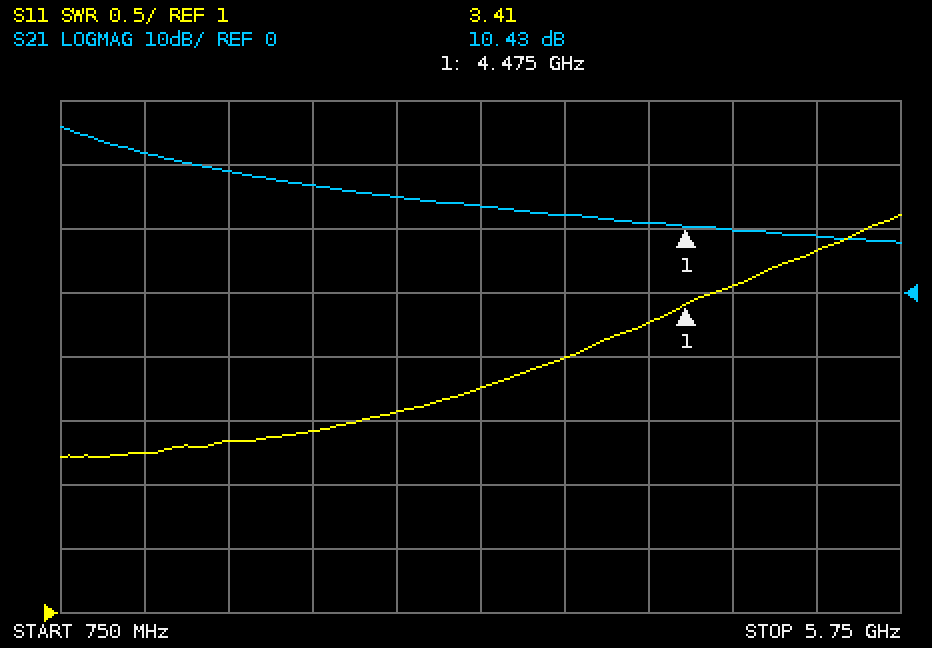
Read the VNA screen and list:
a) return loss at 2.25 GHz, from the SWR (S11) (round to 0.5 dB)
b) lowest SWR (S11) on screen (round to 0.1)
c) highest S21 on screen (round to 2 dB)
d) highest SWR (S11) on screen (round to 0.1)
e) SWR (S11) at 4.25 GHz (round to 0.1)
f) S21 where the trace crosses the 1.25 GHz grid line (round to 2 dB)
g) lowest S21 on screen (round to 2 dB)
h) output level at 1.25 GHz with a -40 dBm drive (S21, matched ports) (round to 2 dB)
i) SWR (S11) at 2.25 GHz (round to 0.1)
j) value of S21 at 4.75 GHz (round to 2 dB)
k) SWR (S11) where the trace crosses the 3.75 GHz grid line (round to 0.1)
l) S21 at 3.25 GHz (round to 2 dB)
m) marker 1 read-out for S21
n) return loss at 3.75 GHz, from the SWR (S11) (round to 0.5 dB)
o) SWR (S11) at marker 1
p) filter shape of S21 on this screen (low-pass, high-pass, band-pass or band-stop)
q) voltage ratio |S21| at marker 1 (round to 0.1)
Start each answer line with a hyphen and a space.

- 7.5 dB
- 2.2
- 26 dB
- 4.1
- 3.3
- 22 dB
- 8 dB
- -18 dBm
- 2.4
- 10 dB
- 3.0
- 14 dB
- 10.43 dB
- 6.0 dB
- 3.41
- low-pass
- 3.3
